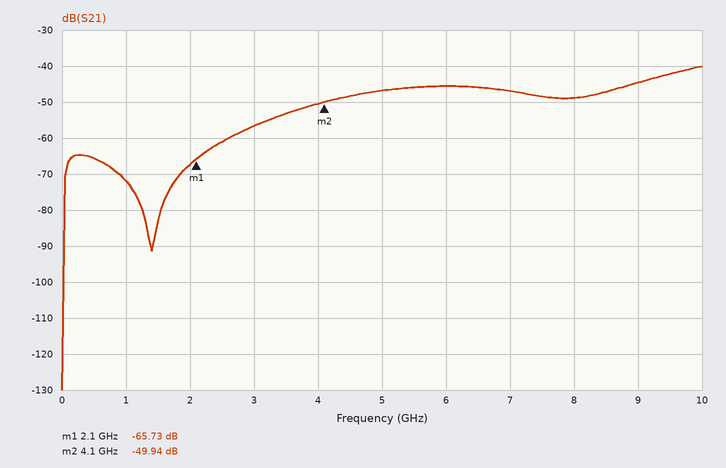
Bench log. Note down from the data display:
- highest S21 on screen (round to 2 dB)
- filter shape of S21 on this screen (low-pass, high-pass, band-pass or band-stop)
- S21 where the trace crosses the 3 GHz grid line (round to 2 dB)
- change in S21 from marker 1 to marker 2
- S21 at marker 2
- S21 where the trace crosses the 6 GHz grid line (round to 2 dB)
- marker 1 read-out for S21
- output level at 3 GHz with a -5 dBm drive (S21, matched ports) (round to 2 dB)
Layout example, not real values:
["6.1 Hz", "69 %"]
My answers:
["-40 dB", "high-pass", "-56 dB", "15.79 dB", "-49.94 dB", "-46 dB", "-65.73 dB", "-62 dBm"]
